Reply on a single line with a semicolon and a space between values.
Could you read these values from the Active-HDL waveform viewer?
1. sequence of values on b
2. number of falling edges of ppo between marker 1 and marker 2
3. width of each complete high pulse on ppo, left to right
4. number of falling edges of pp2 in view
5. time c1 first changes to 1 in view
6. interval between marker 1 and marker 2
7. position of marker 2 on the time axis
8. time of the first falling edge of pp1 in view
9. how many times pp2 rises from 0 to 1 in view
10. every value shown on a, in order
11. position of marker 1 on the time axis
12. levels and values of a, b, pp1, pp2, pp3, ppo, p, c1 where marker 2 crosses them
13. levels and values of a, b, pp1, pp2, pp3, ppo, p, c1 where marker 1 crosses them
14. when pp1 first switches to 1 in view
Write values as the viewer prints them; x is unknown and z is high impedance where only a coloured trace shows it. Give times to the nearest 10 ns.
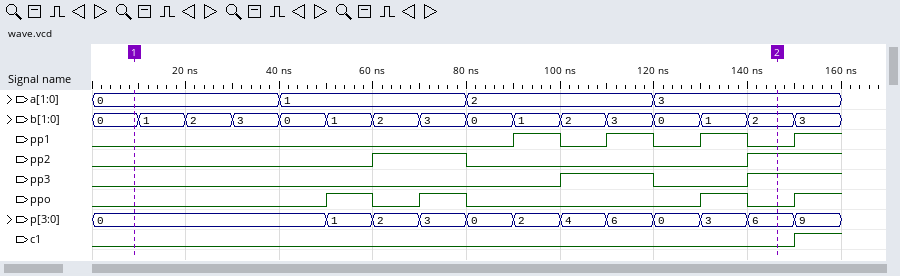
0, 1, 2, 3, 0, 1, 2, 3, 0, 1, 2, 3, 0, 1, 2, 3; 3; 10 ns, 10 ns, 10 ns; 1; 150 ns; 140 ns; 150 ns; 100 ns; 2; 0, 1, 2, 3; 10 ns; a=3, b=2, pp1=0, pp2=1, pp3=1, ppo=0, p=6, c1=0; a=0, b=0, pp1=0, pp2=0, pp3=0, ppo=0, p=0, c1=0; 90 ns
